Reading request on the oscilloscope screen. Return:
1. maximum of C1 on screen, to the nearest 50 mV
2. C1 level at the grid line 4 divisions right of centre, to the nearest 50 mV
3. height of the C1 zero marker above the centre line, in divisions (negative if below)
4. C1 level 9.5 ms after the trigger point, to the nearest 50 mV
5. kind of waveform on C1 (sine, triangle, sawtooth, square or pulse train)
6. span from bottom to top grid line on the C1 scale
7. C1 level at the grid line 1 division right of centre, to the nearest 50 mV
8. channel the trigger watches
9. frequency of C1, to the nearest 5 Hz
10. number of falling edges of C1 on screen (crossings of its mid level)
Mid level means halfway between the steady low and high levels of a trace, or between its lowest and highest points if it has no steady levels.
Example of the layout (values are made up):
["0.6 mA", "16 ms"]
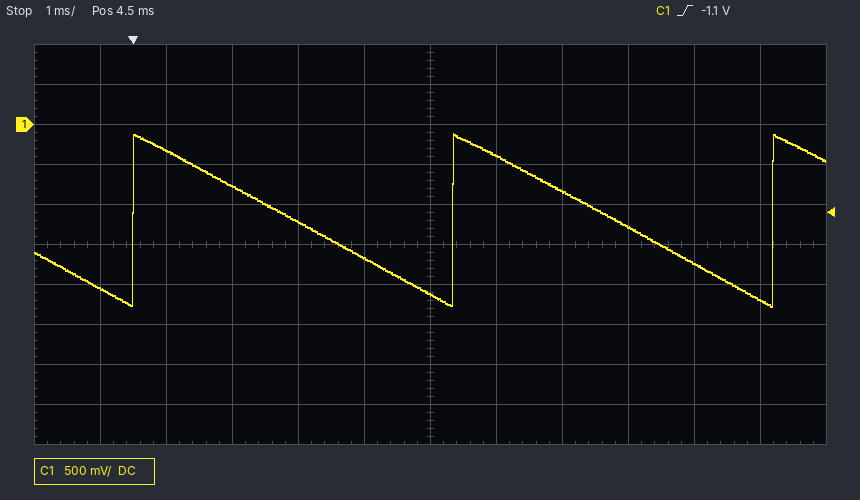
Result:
["-100 mV", "-1.75 V", "+3.0 div", "-2.20 V", "sawtooth", "5 V", "-400 mV", "C1", "205 Hz", "2"]
